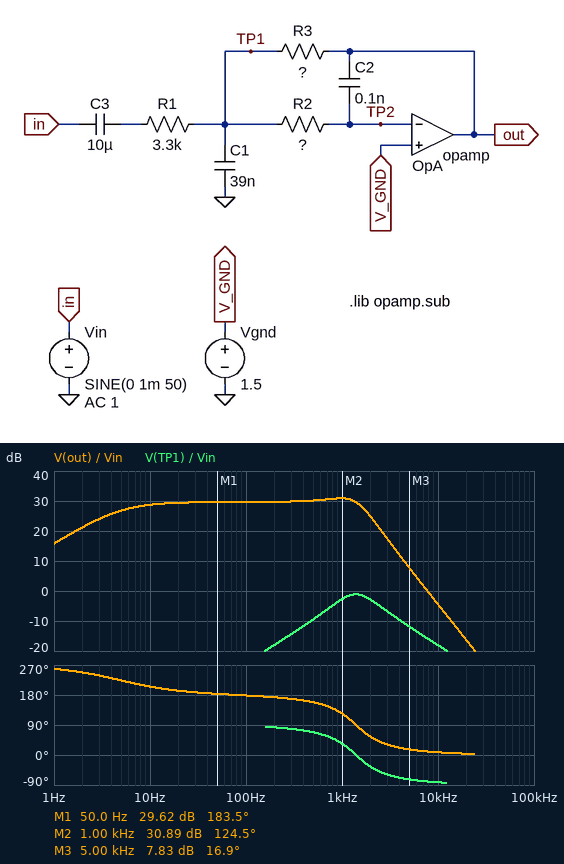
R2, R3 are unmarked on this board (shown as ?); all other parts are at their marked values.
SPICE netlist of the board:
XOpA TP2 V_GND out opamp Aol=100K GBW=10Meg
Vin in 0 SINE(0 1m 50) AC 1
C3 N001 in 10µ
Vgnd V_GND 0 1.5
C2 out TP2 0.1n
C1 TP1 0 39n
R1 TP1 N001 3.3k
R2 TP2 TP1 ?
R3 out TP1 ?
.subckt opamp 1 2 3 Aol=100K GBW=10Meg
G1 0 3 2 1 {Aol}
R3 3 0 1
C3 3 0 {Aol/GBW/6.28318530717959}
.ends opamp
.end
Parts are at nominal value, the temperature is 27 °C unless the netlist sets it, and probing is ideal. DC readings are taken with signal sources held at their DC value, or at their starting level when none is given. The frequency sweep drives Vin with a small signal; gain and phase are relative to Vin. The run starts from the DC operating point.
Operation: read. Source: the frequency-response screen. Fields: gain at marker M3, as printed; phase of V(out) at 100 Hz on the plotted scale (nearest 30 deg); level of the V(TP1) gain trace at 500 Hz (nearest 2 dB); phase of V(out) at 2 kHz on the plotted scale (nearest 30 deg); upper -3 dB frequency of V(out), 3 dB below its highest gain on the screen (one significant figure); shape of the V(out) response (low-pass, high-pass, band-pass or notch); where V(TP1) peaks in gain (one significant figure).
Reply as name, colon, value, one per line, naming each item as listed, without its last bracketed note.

gain at marker M3, as printed: 7.83 dB
phase of V(out) at 100 Hz on the plotted scale: 180 deg
level of the V(TP1) gain trace at 500 Hz: -10 dB
phase of V(out) at 2 kHz on the plotted scale: 60 deg
upper -3 dB frequency of V(out), 3 dB below its highest gain on the screen: 2 kHz
shape of the V(out) response: band-pass
where V(TP1) peaks in gain: 1 kHz
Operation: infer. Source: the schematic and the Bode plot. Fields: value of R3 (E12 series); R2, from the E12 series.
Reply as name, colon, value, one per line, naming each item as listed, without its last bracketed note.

value of R3: 100 kΩ
R2, from the E12 series: 33 kΩ
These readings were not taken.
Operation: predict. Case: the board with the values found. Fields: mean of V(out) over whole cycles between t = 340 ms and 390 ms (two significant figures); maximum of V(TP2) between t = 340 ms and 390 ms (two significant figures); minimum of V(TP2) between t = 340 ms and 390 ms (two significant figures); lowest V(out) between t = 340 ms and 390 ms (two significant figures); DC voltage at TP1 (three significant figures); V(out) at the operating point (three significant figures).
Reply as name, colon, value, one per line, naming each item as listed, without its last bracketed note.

mean of V(out) over whole cycles between t = 340 ms and 390 ms: 1.5 V
maximum of V(TP2) between t = 340 ms and 390 ms: 1.5 V
minimum of V(TP2) between t = 340 ms and 390 ms: 1.5 V
lowest V(out) between t = 340 ms and 390 ms: 1.5 V
DC voltage at TP1: 1.50 V
V(out) at the operating point: 1.50 V
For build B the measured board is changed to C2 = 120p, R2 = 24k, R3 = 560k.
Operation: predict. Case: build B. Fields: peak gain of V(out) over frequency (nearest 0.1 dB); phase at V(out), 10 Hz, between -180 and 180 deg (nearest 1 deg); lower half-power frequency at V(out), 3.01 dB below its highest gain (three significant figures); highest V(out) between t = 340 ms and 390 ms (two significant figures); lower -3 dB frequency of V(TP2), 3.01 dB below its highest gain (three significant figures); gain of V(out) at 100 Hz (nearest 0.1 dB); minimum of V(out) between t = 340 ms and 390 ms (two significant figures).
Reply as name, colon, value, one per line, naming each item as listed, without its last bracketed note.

peak gain of V(out) over frequency: 44.6 dB
phase at V(out), 10 Hz, between -180 and 180 deg: -156 deg
lower half-power frequency at V(out), 3.01 dB below its highest gain: 4.76 Hz
highest V(out) between t = 340 ms and 390 ms: 1.7 V
lower -3 dB frequency of V(TP2), 3.01 dB below its highest gain: 211 Hz
gain of V(out) at 100 Hz: 44.4 dB
minimum of V(out) between t = 340 ms and 390 ms: 1.3 V
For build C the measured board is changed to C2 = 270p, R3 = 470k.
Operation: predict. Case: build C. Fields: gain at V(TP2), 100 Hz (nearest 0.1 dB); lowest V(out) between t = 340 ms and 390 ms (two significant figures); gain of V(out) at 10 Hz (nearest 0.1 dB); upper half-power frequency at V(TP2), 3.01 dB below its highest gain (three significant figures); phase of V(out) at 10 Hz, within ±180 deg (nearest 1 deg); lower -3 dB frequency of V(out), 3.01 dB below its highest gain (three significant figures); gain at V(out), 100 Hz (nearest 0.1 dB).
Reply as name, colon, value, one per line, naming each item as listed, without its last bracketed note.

gain at V(TP2), 100 Hz: -55.9 dB
lowest V(out) between t = 340 ms and 390 ms: 1.4 V
gain of V(out) at 10 Hz: 42.4 dB
upper half-power frequency at V(TP2), 3.01 dB below its highest gain: 1.37 kHz
phase of V(out) at 10 Hz, within ±180 deg: -159 deg
lower -3 dB frequency of V(out), 3.01 dB below its highest gain: 4.64 Hz
gain at V(out), 100 Hz: 41.1 dB
